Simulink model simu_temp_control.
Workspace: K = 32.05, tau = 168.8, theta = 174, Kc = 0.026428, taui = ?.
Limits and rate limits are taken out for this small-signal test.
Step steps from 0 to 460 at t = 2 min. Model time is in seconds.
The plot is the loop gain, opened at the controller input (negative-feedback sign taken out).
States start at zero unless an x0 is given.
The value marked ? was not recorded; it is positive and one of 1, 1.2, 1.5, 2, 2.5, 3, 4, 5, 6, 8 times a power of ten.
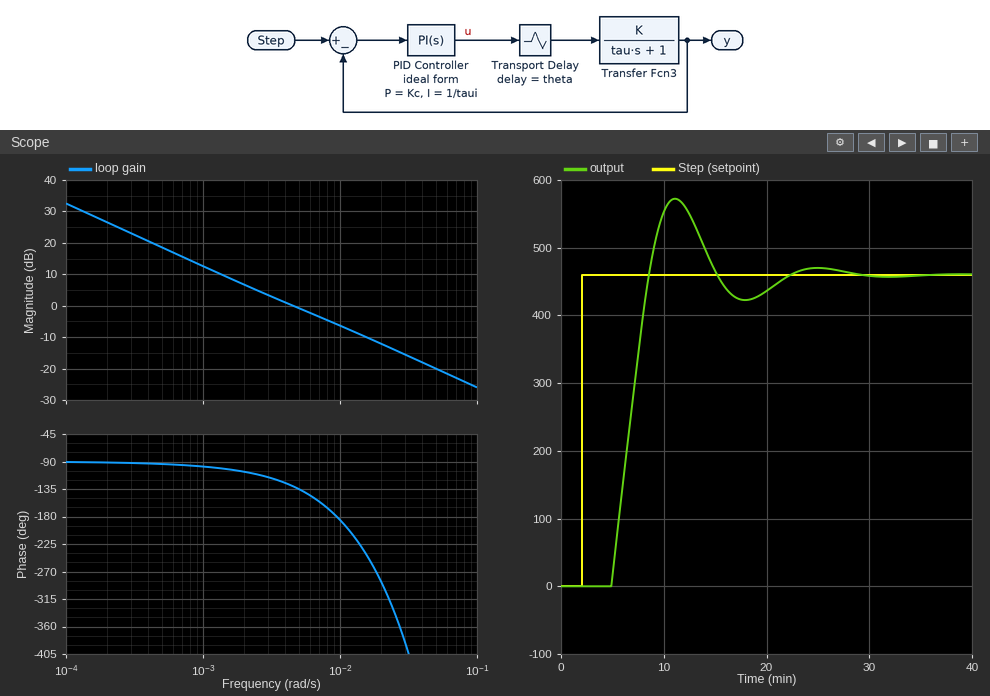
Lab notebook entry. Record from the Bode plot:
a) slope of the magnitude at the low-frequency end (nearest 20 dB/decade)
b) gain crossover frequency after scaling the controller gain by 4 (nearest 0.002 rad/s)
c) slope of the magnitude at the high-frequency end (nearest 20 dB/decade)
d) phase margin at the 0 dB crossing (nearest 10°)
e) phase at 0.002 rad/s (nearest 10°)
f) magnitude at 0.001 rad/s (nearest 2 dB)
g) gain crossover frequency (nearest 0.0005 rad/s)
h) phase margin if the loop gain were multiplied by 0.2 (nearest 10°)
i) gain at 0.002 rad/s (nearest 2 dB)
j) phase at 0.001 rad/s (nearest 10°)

-20 dB/decade
0.020 rad/s
-20 dB/decade
50°
-110°
12 dB
0.0045 rad/s
80°
6 dB
-100°
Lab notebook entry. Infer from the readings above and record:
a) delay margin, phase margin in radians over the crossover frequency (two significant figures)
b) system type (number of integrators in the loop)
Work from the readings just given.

190 s
1
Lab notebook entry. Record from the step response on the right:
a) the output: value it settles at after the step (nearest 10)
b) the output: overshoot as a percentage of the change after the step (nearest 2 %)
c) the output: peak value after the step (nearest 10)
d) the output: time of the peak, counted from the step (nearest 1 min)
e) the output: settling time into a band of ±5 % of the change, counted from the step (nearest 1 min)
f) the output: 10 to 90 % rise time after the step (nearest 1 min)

460
24 %
570
9 min
18 min
3 min
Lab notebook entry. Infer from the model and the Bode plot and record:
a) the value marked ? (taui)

200
